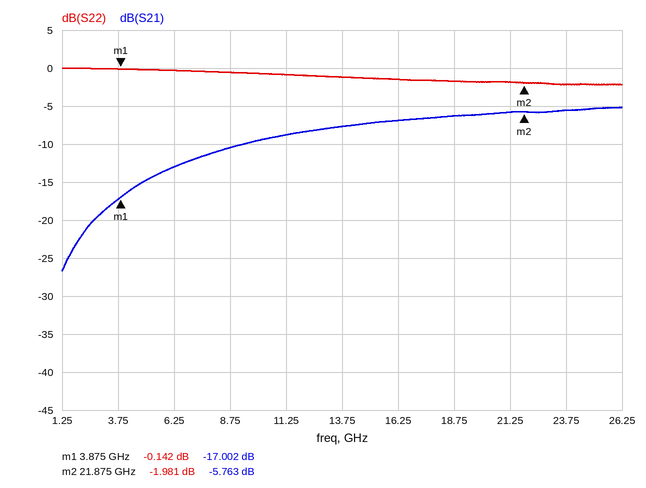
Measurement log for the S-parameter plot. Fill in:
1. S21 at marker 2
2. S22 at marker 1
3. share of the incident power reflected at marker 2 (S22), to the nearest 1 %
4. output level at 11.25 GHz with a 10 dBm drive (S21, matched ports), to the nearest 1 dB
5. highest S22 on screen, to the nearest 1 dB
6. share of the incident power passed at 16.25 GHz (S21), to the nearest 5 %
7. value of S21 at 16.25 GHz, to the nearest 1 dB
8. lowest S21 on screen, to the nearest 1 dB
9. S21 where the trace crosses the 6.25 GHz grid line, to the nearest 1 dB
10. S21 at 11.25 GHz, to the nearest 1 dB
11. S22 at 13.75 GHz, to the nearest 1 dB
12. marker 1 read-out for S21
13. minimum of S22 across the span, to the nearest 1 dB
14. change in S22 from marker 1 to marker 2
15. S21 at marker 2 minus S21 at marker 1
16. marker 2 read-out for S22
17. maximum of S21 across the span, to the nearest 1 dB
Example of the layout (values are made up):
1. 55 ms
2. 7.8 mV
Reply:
1. -5.763 dB
2. -0.142 dB
3. 63 %
4. 1 dBm
5. 0 dB
6. 20 %
7. -7 dB
8. -27 dB
9. -13 dB
10. -9 dB
11. -1 dB
12. -17.002 dB
13. -2 dB
14. -1.839 dB
15. 11.239 dB
16. -1.981 dB
17. -5 dB
